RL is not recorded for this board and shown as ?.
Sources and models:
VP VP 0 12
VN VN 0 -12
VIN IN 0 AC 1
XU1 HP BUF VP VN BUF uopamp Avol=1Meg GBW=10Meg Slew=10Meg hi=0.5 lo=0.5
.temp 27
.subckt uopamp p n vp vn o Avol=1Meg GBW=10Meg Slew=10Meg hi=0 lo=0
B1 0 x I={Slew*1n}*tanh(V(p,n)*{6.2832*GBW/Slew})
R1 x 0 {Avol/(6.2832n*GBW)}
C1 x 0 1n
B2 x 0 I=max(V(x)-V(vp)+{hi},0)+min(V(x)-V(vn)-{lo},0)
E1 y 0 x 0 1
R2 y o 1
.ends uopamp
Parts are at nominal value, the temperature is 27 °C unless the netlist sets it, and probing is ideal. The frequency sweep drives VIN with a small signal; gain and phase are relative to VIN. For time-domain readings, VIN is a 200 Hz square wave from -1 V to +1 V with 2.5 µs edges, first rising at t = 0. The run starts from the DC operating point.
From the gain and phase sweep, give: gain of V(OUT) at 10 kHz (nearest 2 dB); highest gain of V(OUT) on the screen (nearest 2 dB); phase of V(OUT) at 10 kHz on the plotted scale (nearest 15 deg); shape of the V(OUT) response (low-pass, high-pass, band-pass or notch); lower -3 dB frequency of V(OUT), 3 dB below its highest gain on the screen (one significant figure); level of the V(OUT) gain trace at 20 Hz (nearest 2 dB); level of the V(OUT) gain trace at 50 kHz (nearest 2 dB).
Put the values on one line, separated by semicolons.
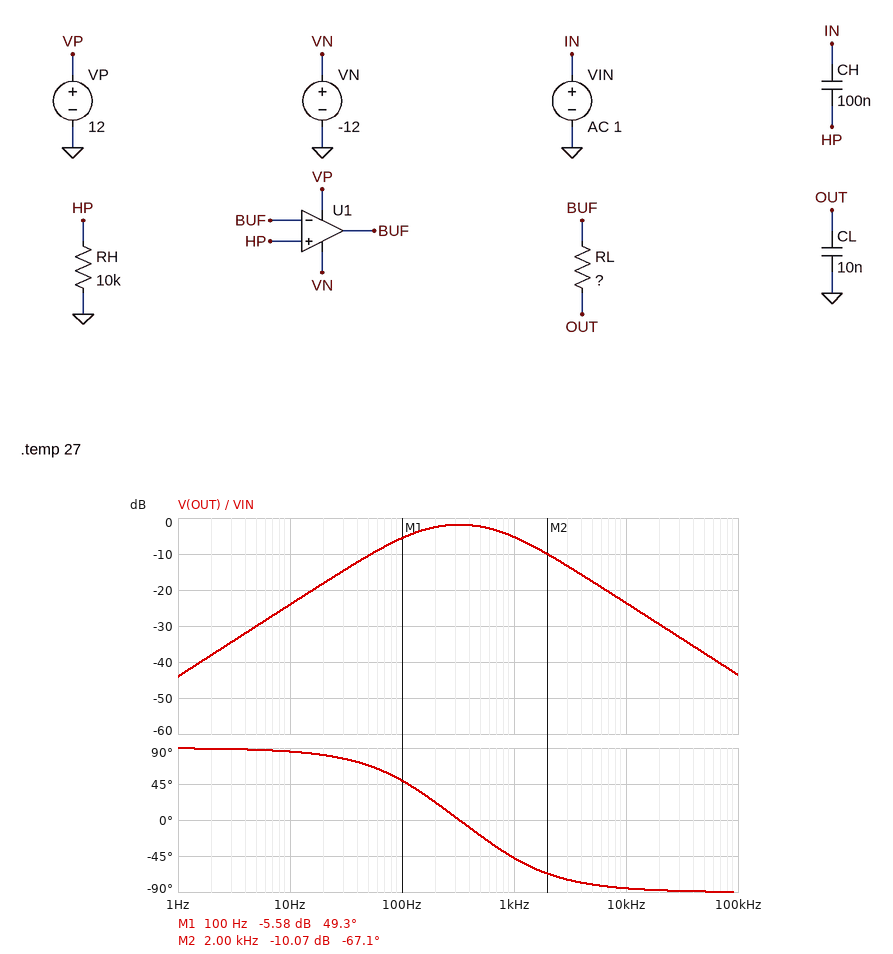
-24 dB; -2 dB; -90 deg; band-pass; 100 Hz; -18 dB; -38 dB
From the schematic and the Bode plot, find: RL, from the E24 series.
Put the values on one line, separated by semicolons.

24 kΩ
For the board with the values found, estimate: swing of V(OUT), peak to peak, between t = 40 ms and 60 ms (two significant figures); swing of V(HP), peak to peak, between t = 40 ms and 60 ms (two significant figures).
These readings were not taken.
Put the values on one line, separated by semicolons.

2.3 V; 3.7 V
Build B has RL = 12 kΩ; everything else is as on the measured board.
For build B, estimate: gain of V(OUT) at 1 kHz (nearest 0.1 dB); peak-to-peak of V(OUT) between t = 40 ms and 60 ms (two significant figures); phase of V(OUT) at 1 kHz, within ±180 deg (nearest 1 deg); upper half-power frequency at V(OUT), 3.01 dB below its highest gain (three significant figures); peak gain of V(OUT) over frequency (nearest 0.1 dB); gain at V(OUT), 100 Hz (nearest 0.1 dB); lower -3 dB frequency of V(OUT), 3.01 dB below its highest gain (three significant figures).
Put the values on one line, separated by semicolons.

-2.1 dB; 2.7 V; -28 deg; 1.62 kHz; -1.0 dB; -5.5 dB; 131 Hz
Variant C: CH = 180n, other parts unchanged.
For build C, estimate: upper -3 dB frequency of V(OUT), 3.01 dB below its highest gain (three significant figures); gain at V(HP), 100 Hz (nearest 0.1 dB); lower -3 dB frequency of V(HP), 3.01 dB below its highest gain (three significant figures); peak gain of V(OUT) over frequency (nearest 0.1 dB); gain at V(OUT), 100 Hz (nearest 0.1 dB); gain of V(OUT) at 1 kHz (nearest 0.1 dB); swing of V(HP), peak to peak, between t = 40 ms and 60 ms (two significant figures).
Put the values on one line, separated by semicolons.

823 Hz; -2.5 dB; 88.4 Hz; -1.1 dB; -2.6 dB; -5.2 dB; 3.2 V
